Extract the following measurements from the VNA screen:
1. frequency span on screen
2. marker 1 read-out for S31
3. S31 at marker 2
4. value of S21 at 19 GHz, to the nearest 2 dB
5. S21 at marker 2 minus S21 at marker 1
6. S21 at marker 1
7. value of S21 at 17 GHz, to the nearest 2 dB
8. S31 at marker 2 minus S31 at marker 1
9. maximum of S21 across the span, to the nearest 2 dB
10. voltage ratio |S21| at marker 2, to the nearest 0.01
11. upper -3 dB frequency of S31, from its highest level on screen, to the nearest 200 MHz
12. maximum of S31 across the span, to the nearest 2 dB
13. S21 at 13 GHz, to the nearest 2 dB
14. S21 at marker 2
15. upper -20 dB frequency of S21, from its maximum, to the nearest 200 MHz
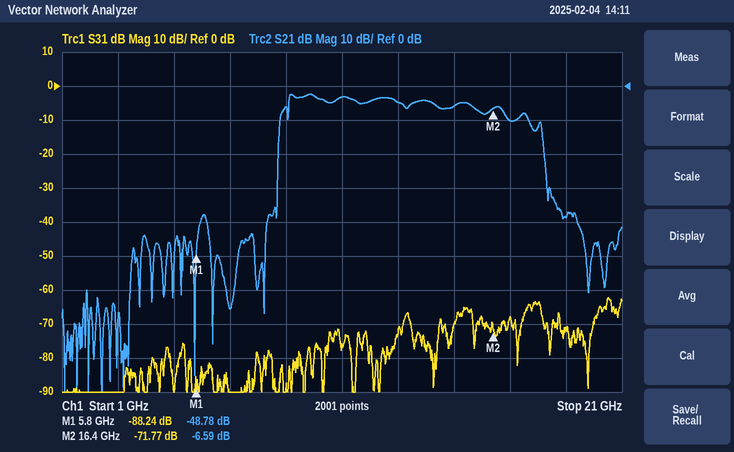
20 GHz
-88.24 dB
-71.77 dB
-38 dB
42.19 dB
-48.78 dB
-10 dB
16.47 dB
-2 dB
0.47
20.6 GHz
-62 dB
-4 dB
-6.59 dB
18.2 GHz
